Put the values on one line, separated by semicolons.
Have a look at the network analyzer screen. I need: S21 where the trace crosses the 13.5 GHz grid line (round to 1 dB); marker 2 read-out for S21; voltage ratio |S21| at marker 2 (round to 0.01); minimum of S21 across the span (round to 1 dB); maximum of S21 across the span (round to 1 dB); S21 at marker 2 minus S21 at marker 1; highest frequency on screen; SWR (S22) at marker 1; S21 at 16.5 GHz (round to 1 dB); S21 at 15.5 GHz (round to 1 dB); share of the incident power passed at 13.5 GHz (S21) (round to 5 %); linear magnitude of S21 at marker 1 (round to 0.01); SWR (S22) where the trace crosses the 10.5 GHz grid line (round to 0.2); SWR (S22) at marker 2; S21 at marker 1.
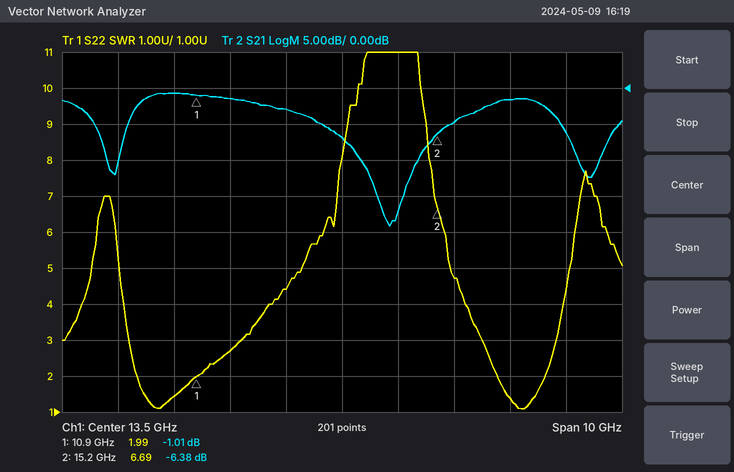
-7 dB; -6.38 dB; 0.48; -19 dB; -1 dB; -5.37 dB; 18.5 GHz; 1.99; -2 dB; -5 dB; 20 %; 0.89; 1.4; 6.69; -1.01 dB
